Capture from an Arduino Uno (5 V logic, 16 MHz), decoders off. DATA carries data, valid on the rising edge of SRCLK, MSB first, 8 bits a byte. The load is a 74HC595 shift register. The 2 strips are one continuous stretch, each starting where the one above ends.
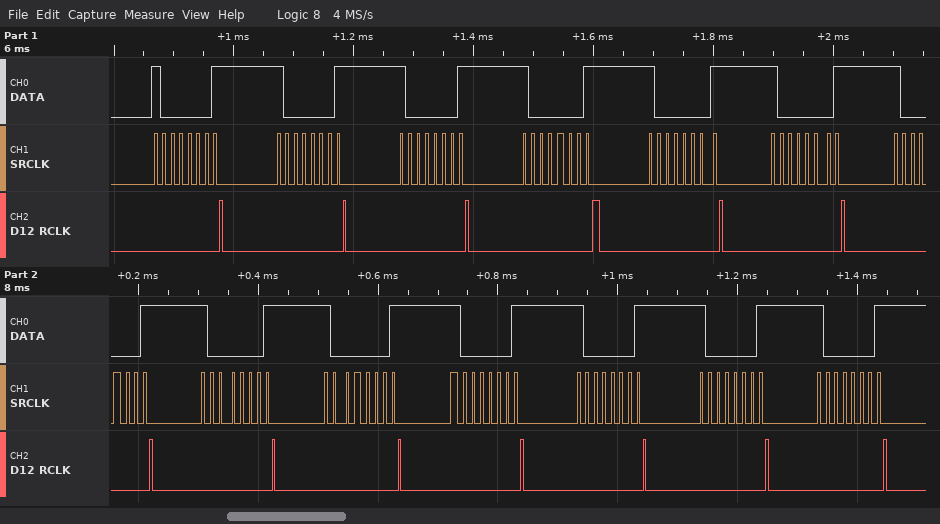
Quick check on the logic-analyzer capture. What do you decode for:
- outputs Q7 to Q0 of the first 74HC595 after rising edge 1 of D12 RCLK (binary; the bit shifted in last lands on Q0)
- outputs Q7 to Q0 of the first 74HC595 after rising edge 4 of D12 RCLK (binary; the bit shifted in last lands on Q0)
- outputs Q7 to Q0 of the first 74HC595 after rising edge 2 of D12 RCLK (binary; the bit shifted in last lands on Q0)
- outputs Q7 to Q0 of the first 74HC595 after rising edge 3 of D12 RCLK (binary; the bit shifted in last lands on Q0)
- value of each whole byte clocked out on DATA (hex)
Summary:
10000001
10000001
10000001
10000001
81 81 81 81 81 81 81 81 81 81 81 81 81
